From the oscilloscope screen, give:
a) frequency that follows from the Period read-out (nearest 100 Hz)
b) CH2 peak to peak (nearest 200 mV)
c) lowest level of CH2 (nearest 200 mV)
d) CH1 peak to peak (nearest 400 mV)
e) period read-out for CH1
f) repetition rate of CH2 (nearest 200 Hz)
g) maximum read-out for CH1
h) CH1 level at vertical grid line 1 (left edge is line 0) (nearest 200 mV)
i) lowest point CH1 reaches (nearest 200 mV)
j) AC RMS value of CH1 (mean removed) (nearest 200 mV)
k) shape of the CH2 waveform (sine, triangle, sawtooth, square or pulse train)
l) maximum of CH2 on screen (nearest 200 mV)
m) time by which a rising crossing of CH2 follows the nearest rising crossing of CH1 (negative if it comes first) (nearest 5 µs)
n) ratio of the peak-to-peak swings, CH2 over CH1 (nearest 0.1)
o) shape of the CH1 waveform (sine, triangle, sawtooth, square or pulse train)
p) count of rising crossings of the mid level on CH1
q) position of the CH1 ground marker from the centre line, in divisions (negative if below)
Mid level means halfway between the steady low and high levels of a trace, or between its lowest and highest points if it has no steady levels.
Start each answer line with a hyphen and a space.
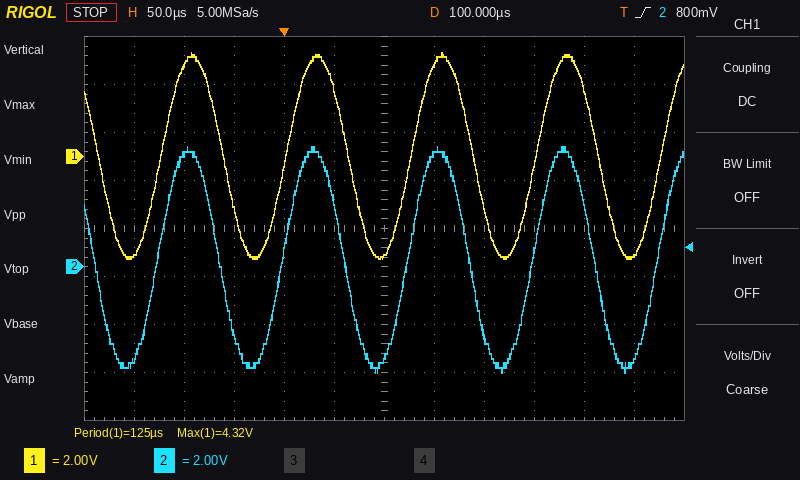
- 8.0 kHz
- 9.4 V
- -4.4 V
- 8.4 V
- 125 µs
- 8.0 kHz
- 4.32 V
- -4.0 V
- -4.2 V
- 3.0 V
- sine
- 5.0 V
- -5 µs
- 1.1
- sine
- 5
- +1.5 div
